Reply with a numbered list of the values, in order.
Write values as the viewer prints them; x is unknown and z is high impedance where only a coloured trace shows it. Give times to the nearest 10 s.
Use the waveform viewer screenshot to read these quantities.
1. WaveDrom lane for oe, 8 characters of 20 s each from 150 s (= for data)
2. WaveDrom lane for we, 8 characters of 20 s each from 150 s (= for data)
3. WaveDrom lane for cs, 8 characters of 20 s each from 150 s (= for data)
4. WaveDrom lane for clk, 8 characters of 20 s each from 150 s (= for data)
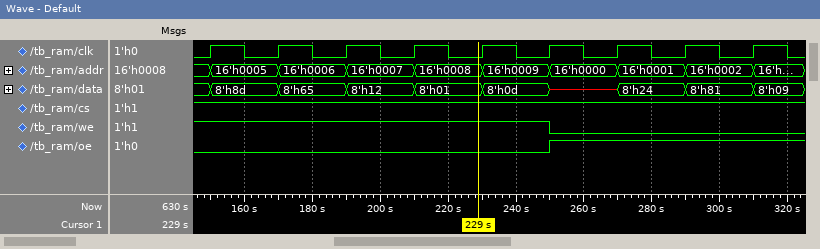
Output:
1. {name: 'oe', wave: '0....1..'}
2. {name: 'we', wave: '1....0..'}
3. {name: 'cs', wave: '1.......'}
4. {name: 'clk', wave: 'p.......'}
